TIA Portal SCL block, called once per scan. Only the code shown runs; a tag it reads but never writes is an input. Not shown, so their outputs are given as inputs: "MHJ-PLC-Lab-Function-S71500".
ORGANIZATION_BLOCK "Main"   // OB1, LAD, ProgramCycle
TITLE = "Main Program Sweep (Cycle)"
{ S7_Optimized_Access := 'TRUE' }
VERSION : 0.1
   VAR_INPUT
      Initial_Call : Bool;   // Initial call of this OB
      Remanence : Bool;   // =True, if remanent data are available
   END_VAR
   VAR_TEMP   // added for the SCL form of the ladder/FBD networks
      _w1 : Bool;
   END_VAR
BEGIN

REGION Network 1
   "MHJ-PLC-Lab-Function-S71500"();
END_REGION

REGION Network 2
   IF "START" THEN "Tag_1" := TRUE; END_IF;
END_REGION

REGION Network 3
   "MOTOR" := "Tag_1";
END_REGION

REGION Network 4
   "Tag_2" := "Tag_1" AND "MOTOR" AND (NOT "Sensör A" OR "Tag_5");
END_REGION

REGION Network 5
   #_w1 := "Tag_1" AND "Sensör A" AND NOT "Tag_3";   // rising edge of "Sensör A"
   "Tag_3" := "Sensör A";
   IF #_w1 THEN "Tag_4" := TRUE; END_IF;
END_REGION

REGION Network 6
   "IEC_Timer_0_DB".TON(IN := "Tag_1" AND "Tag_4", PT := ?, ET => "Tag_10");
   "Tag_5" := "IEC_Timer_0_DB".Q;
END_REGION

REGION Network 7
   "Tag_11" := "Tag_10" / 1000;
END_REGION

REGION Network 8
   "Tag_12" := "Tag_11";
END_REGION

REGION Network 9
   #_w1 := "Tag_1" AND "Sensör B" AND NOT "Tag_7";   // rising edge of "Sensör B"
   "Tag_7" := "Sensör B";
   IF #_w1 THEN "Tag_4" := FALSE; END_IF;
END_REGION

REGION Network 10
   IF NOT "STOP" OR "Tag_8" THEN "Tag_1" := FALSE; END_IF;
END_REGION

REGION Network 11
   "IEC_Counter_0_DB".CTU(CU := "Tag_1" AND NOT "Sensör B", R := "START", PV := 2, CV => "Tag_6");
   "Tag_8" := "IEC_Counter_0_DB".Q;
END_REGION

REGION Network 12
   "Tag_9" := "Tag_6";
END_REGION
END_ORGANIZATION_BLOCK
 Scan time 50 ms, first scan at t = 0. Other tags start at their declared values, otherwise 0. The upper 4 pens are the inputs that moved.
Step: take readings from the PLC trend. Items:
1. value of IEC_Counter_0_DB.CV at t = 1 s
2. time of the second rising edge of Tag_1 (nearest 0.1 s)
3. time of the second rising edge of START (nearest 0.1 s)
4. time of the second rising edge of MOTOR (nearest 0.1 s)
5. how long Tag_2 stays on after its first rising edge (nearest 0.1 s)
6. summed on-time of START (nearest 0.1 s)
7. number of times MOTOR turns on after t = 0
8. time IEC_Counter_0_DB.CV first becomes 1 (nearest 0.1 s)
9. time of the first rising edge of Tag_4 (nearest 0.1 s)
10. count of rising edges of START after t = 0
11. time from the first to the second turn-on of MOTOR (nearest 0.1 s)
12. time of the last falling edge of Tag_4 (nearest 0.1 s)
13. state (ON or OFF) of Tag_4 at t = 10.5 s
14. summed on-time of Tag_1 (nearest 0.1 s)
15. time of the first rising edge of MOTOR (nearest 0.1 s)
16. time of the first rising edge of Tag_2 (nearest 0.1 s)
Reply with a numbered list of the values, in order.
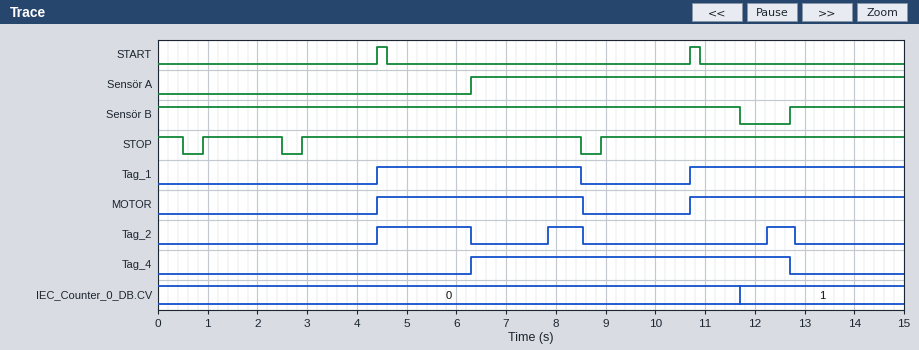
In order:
1. 0
2. 10.7 s
3. 10.7 s
4. 10.7 s
5. 1.9 s
6. 0.4 s
7. 2
8. 11.7 s
9. 6.3 s
10. 2
11. 6.3 s
12. 12.7 s
13. ON
14. 8.4 s
15. 4.4 s
16. 4.4 s
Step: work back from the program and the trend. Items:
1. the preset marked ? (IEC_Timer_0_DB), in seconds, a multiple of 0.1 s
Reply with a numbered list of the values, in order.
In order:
1. 1.5 s
